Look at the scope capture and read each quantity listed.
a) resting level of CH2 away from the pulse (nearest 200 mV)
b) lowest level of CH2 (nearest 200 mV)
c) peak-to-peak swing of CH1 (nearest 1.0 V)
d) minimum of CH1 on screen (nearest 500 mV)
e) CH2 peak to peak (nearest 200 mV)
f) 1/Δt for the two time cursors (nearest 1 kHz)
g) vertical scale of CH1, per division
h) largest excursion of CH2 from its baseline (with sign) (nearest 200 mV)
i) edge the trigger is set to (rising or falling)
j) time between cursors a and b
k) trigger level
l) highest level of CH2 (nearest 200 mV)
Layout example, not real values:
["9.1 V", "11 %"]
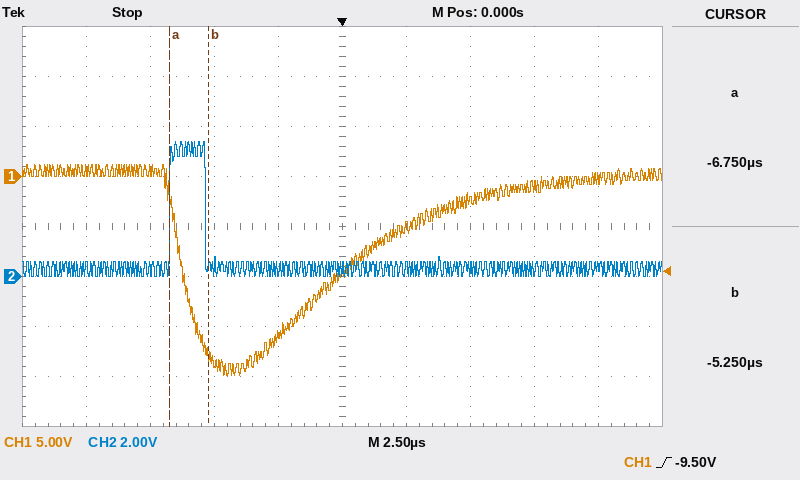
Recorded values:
["400 mV", "0.0 V", "21.0 V", "-20.0 V", "5.4 V", "667 kHz", "5 V", "+5.0 V", "rising", "1.50 µs", "-9.50 V", "5.4 V"]
